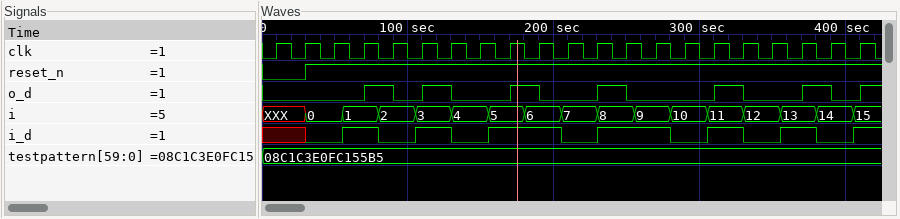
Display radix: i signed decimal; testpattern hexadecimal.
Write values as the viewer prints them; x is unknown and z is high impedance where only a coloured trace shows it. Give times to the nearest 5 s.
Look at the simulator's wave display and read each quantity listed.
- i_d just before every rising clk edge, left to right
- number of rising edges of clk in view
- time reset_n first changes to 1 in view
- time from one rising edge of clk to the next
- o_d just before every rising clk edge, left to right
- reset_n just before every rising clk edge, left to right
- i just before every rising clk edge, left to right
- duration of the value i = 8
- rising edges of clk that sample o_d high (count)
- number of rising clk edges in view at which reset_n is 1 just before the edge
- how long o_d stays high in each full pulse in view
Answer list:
x x 0 1 0 1 1 0 1 1 0 0 1 1 0 1 1 0 1 0 1
21
30 s
20 s
0 0 0 0 1 0 1 0 0 1 0 0 1 0 0 0 1 0 0 1 0
0 0 1 1 1 1 1 1 1 1 1 1 1 1 1 1 1 1 1 1 1
XXX, XXX, 0, 1, 2, 3, 3, 4, 5, 6, 7, 7, 8, 9, 10, 11, 11, 12, 13, 14, 15
25 s
6
19
20 s, 20 s, 20 s, 20 s, 20 s, 20 s
